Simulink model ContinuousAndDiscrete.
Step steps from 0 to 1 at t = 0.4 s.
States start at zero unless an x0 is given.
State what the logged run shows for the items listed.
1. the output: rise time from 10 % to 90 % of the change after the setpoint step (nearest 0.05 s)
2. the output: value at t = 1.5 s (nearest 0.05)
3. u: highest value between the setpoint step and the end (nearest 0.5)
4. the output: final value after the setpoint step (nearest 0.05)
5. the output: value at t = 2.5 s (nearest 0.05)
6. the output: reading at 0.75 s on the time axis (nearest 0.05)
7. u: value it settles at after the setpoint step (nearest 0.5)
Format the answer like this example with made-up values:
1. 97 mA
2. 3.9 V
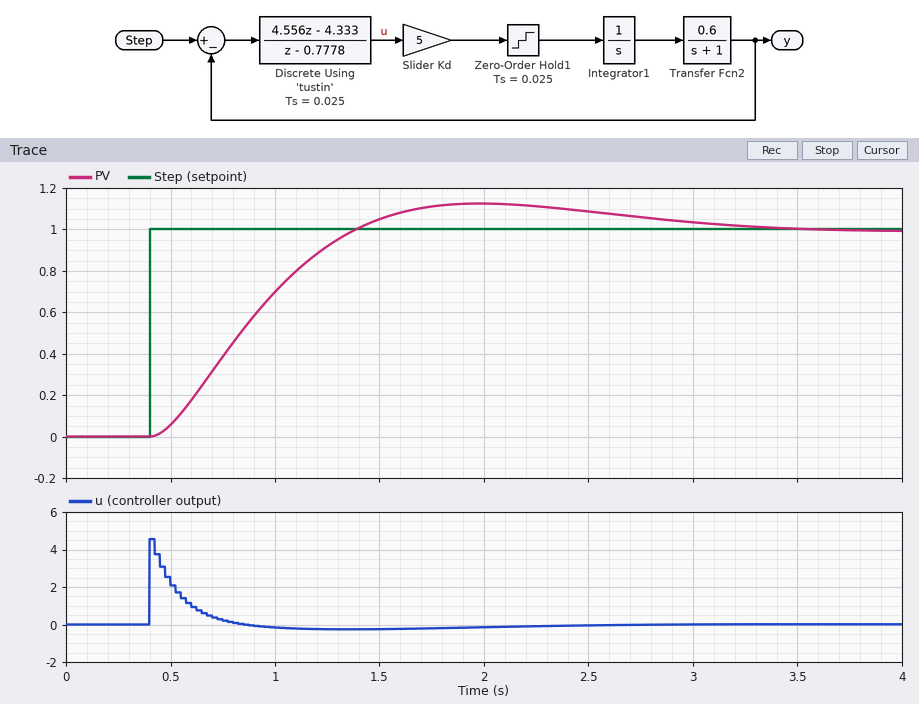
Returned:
1. 0.70 s
2. 1.05
3. 4.5
4. 1.00
5. 1.10
6. 0.40
7. 0.0
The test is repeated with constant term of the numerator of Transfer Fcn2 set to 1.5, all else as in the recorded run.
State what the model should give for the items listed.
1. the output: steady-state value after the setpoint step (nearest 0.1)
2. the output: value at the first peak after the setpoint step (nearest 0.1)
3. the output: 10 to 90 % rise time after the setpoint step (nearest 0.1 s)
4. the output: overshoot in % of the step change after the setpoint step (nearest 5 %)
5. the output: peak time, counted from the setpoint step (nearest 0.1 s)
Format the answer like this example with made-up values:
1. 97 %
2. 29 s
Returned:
1. 1.0
2. 1.2
3. 0.3 s
4. 20 %
5. 0.7 s
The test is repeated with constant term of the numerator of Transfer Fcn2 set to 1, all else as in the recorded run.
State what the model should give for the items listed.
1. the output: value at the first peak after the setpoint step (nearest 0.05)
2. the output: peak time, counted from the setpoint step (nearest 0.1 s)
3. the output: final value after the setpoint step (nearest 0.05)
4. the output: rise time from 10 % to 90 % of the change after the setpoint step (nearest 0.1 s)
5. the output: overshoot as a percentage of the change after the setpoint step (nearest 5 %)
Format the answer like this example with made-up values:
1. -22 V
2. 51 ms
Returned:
1. 1.15
2. 1.0 s
3. 1.00
4. 0.4 s
5. 15 %
